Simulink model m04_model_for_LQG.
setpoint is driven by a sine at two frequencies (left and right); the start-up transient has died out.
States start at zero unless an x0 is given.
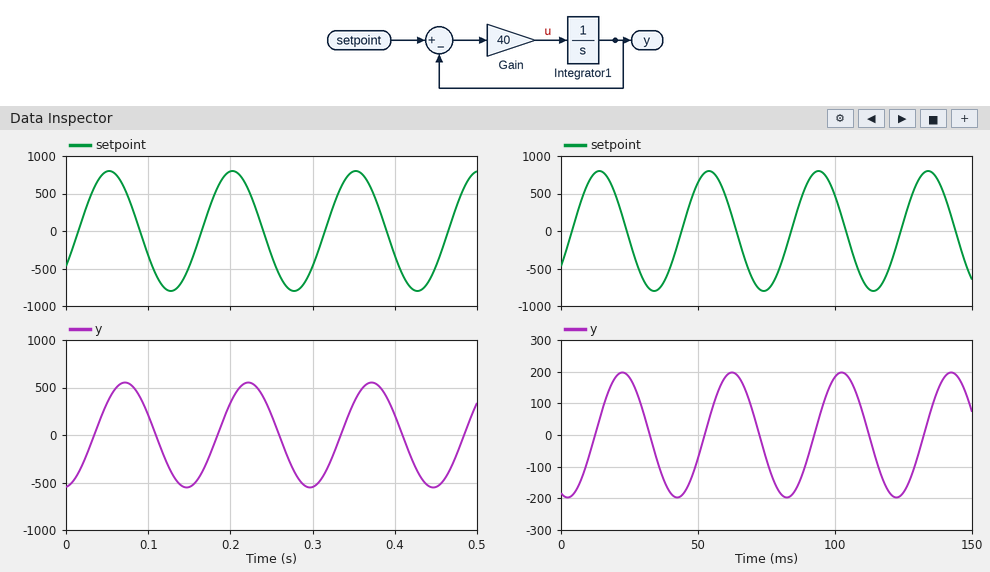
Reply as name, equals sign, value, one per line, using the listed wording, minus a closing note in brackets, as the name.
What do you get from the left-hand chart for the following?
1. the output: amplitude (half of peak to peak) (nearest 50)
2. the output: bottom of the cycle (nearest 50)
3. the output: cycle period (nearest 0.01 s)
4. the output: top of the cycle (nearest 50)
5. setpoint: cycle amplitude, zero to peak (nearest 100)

the output: amplitude (half of peak to peak) = 550
the output: bottom of the cycle = -550
the output: cycle period = 0.15 s
the output: top of the cycle = 550
setpoint: cycle amplitude, zero to peak = 800
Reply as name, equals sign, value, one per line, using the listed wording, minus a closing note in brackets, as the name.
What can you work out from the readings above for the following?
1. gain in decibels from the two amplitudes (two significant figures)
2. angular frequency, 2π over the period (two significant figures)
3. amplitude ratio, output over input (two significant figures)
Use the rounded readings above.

gain in decibels from the two amplitudes = -3.3 dB
angular frequency, 2π over the period = 42 rad/s
amplitude ratio, output over input = 0.69
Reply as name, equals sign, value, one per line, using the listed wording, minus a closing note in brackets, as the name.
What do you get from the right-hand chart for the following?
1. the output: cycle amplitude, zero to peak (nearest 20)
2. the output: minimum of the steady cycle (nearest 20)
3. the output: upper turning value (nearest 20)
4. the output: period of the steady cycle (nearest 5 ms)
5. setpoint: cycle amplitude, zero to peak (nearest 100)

the output: cycle amplitude, zero to peak = 200
the output: minimum of the steady cycle = -200
the output: upper turning value = 200
the output: period of the steady cycle = 40 ms
setpoint: cycle amplitude, zero to peak = 800
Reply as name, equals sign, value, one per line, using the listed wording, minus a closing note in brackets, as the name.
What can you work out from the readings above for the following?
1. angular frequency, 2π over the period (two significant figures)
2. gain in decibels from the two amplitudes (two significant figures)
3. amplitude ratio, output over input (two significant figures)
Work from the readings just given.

angular frequency, 2π over the period = 0.16 rad/ms
gain in decibels from the two amplitudes = -12 dB
amplitude ratio, output over input = 0.25
